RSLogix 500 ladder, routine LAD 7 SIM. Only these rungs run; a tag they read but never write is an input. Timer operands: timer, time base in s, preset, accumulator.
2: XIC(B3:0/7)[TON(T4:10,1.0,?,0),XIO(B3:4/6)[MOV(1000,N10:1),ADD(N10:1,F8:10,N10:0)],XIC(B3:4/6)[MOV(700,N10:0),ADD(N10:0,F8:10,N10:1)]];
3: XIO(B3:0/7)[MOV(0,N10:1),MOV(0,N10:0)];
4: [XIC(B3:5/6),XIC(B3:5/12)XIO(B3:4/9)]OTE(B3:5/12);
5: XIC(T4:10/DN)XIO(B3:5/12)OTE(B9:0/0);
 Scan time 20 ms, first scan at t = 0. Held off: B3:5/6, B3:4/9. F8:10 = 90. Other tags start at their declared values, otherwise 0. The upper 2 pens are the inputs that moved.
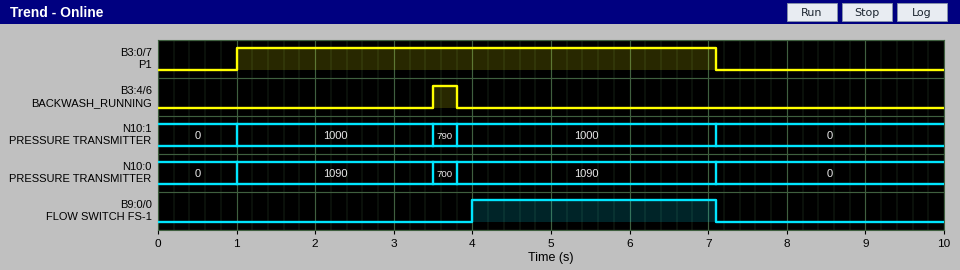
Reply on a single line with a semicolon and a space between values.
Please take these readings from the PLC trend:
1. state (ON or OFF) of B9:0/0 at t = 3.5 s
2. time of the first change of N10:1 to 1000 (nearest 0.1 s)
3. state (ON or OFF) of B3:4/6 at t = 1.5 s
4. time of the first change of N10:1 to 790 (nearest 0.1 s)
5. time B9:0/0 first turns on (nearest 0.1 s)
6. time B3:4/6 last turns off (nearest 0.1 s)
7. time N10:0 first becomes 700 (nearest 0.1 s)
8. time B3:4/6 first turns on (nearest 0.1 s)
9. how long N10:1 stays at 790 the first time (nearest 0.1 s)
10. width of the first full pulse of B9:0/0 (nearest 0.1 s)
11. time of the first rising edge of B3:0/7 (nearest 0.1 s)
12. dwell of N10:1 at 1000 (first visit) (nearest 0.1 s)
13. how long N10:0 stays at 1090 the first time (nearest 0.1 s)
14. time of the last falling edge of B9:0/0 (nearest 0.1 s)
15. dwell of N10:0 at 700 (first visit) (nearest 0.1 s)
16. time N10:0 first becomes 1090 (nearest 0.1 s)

OFF; 1.0 s; OFF; 3.5 s; 4.0 s; 3.8 s; 3.5 s; 3.5 s; 0.3 s; 3.1 s; 1.0 s; 2.5 s; 2.5 s; 7.1 s; 0.3 s; 1.0 s
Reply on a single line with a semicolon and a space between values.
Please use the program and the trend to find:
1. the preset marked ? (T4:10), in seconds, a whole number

3 s
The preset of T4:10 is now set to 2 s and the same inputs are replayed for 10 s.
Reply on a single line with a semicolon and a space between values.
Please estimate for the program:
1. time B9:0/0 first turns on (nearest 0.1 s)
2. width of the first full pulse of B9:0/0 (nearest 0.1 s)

3.0 s; 4.1 s
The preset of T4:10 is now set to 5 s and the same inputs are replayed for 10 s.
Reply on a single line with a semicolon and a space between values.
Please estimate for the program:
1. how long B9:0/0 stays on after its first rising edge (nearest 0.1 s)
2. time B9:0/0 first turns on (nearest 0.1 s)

1.1 s; 6.0 s
